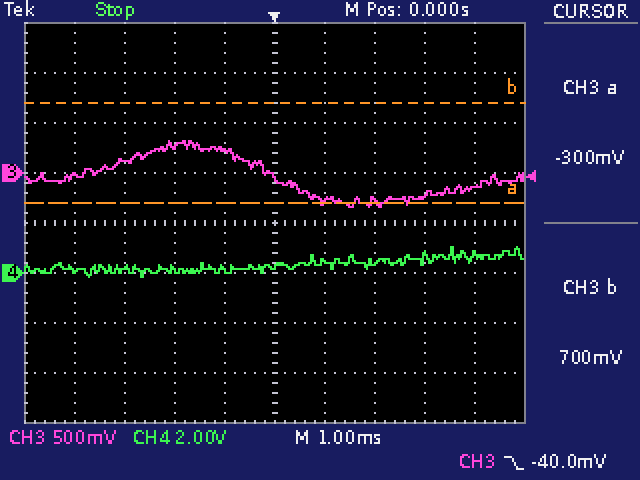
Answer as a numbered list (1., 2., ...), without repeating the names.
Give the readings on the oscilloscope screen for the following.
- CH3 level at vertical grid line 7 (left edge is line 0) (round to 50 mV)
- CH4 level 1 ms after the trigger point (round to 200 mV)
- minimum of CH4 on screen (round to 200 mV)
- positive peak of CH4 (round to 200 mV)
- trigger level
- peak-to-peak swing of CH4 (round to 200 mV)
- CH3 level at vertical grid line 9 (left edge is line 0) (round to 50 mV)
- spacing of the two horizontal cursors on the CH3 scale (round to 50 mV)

1. -300 mV
2. 400 mV
3. -200 mV
4. 1.0 V
5. -40.0 mV
6. 1.2 V
7. -150 mV
8. 1.00 V
